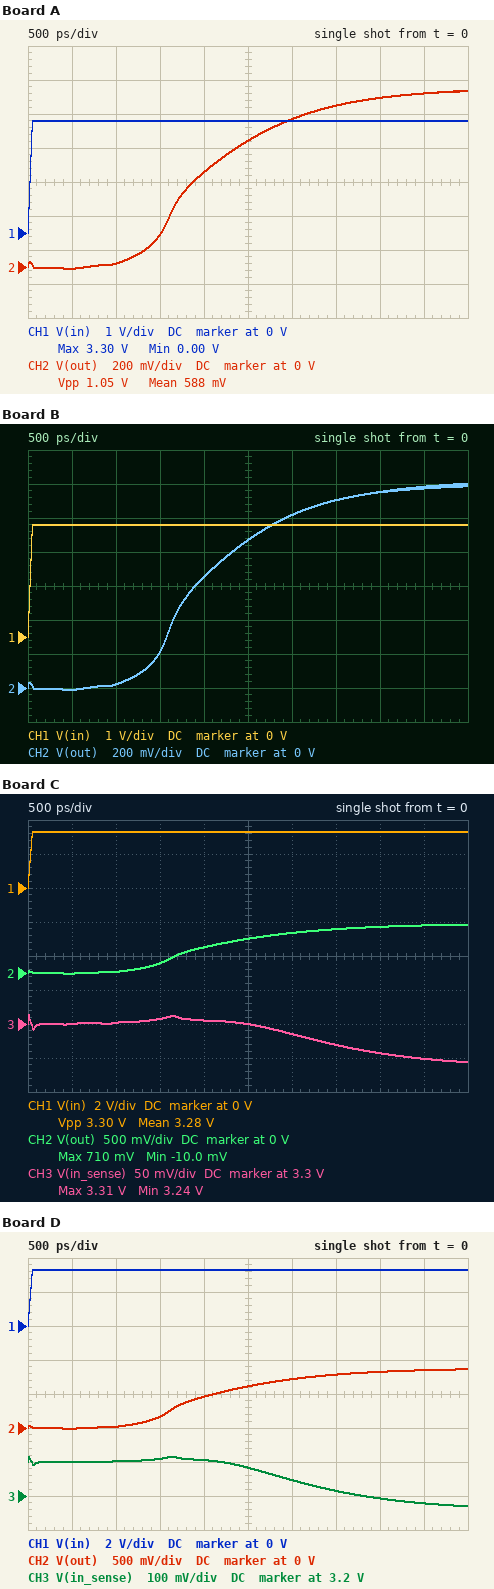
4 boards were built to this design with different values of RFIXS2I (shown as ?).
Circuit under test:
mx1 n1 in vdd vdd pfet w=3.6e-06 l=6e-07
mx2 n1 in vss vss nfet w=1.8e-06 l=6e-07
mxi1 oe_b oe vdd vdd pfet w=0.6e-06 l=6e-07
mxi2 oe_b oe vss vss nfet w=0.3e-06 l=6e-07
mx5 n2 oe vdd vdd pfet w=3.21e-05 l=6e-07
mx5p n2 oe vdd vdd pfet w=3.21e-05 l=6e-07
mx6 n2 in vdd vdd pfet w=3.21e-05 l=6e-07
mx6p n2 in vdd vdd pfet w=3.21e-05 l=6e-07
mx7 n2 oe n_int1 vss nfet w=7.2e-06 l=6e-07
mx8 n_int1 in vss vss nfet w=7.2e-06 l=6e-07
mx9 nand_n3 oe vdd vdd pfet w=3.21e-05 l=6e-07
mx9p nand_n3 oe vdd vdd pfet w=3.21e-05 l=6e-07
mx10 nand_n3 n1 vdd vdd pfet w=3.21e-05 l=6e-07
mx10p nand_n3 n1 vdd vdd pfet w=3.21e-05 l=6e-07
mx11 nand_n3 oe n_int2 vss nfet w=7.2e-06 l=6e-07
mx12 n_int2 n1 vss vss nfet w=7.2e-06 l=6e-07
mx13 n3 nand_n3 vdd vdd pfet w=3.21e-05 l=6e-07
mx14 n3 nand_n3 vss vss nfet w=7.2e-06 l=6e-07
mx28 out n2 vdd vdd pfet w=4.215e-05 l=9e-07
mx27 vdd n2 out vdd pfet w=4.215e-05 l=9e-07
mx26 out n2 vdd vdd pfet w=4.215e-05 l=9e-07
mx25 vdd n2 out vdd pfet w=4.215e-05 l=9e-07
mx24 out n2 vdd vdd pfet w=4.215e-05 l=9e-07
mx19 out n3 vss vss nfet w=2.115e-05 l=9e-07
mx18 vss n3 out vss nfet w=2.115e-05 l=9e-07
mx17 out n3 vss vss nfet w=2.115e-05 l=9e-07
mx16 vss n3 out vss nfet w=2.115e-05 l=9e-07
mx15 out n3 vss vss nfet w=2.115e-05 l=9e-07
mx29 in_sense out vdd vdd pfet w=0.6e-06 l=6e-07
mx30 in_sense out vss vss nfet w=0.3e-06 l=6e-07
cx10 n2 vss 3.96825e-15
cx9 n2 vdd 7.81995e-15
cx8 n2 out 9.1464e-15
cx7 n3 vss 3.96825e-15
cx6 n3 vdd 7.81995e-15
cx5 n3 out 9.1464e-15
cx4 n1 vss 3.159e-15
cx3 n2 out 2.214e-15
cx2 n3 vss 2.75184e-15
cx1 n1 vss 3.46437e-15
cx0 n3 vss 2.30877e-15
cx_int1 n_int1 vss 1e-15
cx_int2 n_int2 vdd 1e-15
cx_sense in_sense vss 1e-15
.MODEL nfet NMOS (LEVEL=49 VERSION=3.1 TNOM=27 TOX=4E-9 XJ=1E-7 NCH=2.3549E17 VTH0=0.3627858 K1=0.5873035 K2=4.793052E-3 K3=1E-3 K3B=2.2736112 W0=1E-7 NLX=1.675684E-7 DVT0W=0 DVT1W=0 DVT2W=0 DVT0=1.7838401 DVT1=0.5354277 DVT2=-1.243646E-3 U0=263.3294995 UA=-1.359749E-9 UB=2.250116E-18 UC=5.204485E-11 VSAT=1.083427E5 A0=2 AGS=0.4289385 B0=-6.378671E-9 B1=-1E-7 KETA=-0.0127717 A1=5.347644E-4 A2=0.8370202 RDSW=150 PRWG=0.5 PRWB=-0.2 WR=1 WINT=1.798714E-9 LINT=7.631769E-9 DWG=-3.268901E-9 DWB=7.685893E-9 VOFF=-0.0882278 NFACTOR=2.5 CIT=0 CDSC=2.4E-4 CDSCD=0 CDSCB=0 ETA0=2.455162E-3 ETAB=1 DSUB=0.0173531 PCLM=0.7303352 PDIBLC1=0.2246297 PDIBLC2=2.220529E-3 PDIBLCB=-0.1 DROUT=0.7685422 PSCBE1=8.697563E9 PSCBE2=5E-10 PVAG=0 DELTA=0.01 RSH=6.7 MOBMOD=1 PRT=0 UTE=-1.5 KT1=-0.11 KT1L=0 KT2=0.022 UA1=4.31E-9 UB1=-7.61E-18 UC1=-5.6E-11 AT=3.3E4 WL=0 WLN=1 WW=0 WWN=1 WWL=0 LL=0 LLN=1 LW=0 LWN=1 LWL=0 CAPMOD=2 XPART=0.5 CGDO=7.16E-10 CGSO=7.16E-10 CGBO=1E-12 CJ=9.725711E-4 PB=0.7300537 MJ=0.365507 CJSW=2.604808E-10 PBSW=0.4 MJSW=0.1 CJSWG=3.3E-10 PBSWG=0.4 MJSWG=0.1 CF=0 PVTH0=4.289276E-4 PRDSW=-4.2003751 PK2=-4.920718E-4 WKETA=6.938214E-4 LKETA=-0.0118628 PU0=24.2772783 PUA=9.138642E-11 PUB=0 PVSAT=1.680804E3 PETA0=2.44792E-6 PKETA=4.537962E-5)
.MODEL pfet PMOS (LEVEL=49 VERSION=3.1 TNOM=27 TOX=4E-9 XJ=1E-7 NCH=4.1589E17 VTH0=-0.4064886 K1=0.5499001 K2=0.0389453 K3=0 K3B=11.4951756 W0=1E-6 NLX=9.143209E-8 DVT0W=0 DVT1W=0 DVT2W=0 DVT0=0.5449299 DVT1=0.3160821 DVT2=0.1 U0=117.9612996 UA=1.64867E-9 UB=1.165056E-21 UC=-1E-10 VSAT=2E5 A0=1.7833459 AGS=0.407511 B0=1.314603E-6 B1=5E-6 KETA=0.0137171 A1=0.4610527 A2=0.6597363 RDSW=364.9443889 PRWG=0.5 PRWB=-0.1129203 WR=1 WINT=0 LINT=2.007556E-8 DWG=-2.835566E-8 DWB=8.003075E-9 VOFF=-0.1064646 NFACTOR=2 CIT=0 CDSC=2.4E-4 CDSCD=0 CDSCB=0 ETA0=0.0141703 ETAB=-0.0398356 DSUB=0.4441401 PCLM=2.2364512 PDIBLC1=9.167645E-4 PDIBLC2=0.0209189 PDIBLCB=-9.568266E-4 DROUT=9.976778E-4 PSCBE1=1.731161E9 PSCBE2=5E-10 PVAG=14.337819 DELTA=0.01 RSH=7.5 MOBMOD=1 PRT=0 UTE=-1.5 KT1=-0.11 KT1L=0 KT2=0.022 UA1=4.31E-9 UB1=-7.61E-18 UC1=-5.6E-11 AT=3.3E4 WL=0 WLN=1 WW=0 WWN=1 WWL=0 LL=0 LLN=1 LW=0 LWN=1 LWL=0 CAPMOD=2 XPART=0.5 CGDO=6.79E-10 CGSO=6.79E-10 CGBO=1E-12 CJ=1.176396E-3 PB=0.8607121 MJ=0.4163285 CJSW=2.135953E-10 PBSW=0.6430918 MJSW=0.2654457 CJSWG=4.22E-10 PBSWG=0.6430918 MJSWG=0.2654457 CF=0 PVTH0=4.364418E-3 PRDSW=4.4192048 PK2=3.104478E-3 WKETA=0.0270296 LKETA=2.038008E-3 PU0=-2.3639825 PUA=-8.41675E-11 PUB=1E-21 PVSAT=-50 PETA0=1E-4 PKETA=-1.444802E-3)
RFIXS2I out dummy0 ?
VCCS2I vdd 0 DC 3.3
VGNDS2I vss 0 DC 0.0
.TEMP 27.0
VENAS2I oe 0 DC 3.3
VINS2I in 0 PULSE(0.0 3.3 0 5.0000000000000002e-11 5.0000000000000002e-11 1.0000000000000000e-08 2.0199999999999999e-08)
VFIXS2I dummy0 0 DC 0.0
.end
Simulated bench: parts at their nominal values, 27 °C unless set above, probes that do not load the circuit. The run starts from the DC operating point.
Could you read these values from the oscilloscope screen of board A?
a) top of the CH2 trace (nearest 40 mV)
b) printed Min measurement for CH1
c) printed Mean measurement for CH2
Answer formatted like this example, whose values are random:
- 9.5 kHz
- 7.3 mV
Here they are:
- 1.04 V
- 0.00 V
- 588 mV
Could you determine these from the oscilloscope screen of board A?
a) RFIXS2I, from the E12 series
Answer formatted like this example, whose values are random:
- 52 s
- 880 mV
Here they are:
- 33 Ω
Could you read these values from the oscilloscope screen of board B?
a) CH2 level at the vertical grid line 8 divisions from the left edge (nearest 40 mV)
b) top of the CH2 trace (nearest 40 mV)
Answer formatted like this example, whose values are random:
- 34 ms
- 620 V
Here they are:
- 1.16 V
- 1.20 V
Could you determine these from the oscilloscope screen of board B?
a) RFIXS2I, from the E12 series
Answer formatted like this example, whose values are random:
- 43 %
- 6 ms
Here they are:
- 39 Ω
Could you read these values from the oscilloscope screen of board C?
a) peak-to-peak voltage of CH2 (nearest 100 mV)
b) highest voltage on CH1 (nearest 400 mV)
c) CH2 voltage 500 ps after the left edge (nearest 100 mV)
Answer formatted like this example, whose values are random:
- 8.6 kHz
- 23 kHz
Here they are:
- 700 mV
- 3.2 V
- 0 V
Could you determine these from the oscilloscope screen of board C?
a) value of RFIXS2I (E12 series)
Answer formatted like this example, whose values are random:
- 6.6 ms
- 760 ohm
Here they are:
- 22 Ω
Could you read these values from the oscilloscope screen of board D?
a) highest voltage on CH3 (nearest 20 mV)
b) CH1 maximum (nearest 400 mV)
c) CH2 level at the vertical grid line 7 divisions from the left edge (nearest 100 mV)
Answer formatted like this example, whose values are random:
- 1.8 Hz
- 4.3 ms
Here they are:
- 3.32 V
- 3.2 V
- 800 mV
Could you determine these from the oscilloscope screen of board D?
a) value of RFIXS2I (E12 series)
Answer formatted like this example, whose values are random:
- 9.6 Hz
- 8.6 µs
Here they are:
- 27 Ω
